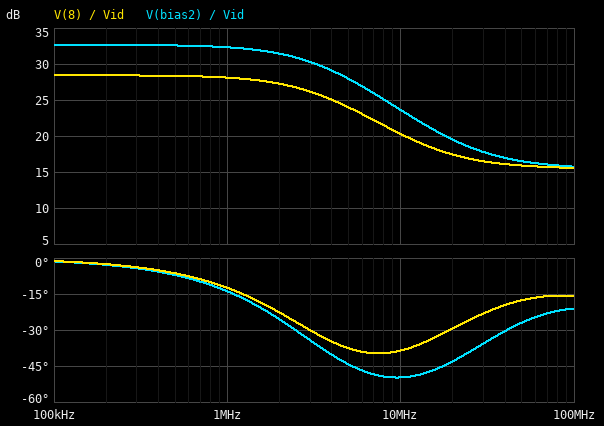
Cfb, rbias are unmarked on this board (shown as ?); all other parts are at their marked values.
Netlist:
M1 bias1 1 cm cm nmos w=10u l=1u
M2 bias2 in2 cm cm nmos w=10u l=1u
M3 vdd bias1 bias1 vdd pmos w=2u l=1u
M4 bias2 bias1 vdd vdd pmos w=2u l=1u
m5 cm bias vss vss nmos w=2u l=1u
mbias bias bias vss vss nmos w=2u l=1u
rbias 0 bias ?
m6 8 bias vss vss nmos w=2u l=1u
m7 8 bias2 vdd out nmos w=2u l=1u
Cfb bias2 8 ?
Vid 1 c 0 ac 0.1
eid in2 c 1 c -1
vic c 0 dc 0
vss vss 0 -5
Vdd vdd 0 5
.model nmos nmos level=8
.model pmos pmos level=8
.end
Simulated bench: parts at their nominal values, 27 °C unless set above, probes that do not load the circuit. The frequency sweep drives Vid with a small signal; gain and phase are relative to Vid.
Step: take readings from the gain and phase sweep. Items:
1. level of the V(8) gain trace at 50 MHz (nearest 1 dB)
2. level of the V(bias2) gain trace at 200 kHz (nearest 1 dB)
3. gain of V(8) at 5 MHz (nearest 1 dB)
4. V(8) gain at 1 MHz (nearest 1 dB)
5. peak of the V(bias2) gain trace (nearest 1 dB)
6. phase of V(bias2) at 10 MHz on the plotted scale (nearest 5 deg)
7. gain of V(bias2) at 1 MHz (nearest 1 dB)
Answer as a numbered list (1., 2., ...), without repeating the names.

1. 16 dB
2. 33 dB
3. 24 dB
4. 28 dB
5. 33 dB
6. -50 deg
7. 32 dB
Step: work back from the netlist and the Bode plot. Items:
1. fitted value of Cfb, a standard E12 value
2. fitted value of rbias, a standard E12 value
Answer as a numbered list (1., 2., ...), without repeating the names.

1. 5.6 pF
2. 82 kΩ
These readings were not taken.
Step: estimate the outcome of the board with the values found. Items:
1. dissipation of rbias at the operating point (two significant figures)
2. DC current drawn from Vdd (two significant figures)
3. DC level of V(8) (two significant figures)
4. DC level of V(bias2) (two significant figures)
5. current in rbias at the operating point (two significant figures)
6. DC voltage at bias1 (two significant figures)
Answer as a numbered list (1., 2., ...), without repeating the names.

1. 240 µW
2. 840 µA
3. 2.3 V
4. 4.1 V
5. 54 µA
6. 4.1 V
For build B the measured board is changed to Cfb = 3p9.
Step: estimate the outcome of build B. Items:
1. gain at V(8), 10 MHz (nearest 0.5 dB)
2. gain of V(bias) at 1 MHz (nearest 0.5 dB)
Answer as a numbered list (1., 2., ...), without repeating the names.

1. 22.0 dB
2. -58.0 dB
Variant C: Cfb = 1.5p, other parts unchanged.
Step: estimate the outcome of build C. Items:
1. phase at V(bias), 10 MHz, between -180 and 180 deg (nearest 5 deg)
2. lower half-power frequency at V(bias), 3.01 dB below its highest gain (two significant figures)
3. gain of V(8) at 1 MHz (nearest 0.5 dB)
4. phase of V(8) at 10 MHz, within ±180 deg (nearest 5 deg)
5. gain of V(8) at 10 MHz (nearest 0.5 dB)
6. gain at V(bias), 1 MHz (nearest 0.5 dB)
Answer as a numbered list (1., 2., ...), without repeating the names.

1. 60 deg
2. 300 MHz
3. 28.5 dB
4. -30 deg
5. 26.5 dB
6. -58.0 dB
